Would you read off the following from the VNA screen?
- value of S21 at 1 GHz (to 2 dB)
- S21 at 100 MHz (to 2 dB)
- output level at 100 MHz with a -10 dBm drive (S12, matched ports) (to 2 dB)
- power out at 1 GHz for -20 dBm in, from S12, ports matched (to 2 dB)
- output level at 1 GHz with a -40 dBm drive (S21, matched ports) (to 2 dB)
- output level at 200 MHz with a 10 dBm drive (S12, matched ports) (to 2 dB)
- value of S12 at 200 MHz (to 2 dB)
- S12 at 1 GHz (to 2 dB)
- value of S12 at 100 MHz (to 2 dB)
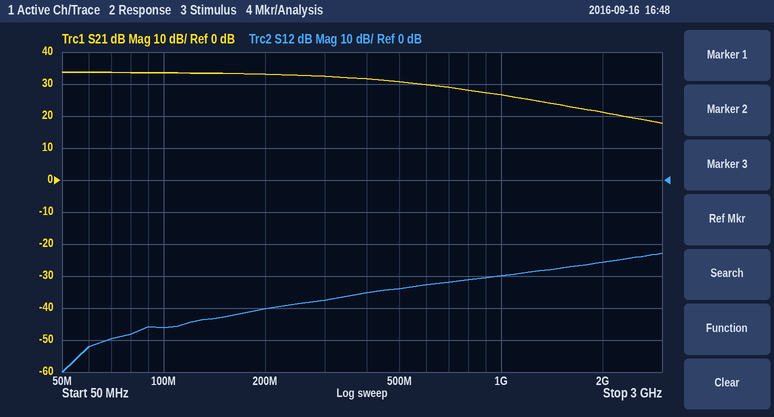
26 dB
34 dB
-56 dBm
-50 dBm
-14 dBm
-30 dBm
-40 dB
-30 dB
-46 dB
